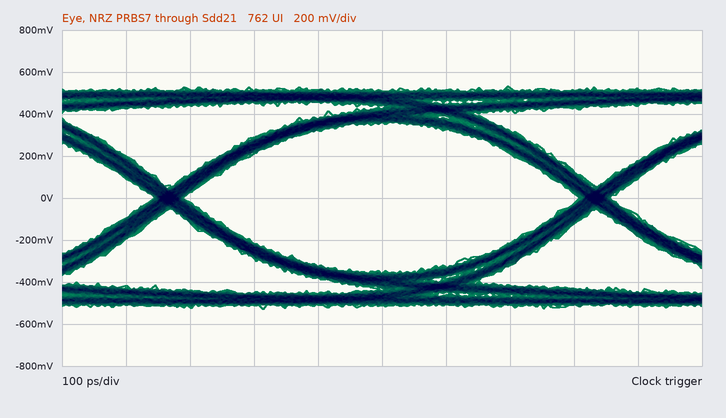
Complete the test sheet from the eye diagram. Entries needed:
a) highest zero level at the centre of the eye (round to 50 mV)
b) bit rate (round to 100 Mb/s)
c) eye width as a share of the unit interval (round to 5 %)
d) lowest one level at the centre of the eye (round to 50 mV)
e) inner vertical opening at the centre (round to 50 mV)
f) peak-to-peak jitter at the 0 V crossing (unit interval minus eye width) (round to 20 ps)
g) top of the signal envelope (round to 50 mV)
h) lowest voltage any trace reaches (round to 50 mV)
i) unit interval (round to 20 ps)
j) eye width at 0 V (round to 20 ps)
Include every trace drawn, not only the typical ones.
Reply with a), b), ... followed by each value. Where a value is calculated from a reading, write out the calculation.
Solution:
a) -350 mV
b) 1.5 Gb/s
c) 620 ps / 660 ps ≈ 93.9 %, so 95 % to the nearest 5 %
d) 350 mV
e) 700 mV
f) 40 ps
g) 550 mV
h) -550 mV
i) 660 ps
j) 620 ps
